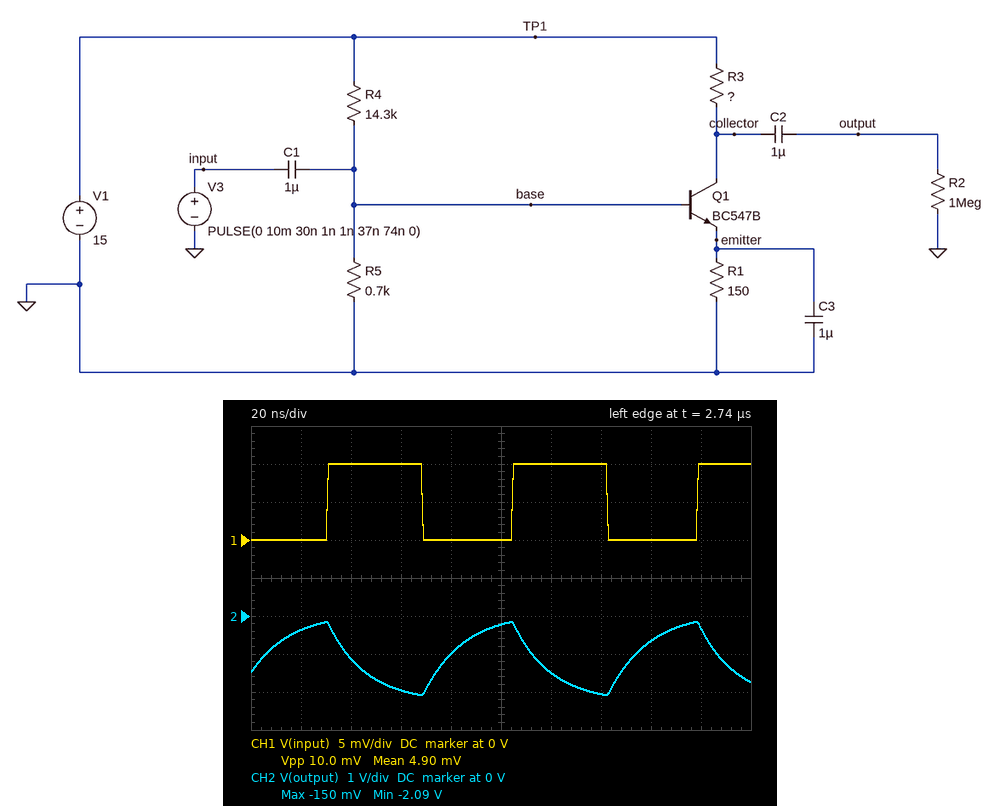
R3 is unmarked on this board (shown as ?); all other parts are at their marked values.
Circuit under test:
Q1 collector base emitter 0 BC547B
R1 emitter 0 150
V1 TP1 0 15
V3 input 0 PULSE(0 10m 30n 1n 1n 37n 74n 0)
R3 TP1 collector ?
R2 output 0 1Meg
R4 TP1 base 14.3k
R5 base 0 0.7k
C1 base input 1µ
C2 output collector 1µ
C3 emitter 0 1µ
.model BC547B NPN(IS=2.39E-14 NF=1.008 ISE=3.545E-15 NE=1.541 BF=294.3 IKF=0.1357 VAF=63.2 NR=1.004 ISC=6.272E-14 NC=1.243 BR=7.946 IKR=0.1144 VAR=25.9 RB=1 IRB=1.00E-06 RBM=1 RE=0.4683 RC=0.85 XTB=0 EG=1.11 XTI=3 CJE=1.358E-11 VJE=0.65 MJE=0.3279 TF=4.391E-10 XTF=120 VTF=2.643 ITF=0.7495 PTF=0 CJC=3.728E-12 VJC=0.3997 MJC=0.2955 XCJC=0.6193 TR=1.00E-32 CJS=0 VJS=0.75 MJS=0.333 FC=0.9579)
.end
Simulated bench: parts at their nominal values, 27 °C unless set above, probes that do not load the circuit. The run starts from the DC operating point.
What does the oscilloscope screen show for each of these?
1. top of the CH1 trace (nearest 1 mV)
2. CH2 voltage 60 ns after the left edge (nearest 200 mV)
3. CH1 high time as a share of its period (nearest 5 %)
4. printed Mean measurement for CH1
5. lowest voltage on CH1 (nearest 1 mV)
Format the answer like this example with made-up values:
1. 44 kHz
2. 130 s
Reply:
1. 10 mV
2. -2.0 V
3. 50 %
4. 4.90 mV
5. 0 V
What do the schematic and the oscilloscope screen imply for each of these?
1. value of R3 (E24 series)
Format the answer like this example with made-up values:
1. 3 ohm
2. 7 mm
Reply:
1. 11 kΩ
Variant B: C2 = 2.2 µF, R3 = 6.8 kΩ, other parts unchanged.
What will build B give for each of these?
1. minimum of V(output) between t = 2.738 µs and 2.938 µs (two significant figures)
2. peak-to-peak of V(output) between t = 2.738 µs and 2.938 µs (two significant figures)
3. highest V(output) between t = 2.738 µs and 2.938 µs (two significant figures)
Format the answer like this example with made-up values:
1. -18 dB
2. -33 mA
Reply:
1. -1.5 V
2. 1.5 V
3. 14 mV
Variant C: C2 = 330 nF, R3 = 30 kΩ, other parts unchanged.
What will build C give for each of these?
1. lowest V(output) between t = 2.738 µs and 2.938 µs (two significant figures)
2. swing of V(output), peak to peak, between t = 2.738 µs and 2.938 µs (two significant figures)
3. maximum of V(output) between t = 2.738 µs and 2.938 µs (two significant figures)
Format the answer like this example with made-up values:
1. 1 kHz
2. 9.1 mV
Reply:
1. -62 mV
2. 56 mV
3. -6.2 mV
